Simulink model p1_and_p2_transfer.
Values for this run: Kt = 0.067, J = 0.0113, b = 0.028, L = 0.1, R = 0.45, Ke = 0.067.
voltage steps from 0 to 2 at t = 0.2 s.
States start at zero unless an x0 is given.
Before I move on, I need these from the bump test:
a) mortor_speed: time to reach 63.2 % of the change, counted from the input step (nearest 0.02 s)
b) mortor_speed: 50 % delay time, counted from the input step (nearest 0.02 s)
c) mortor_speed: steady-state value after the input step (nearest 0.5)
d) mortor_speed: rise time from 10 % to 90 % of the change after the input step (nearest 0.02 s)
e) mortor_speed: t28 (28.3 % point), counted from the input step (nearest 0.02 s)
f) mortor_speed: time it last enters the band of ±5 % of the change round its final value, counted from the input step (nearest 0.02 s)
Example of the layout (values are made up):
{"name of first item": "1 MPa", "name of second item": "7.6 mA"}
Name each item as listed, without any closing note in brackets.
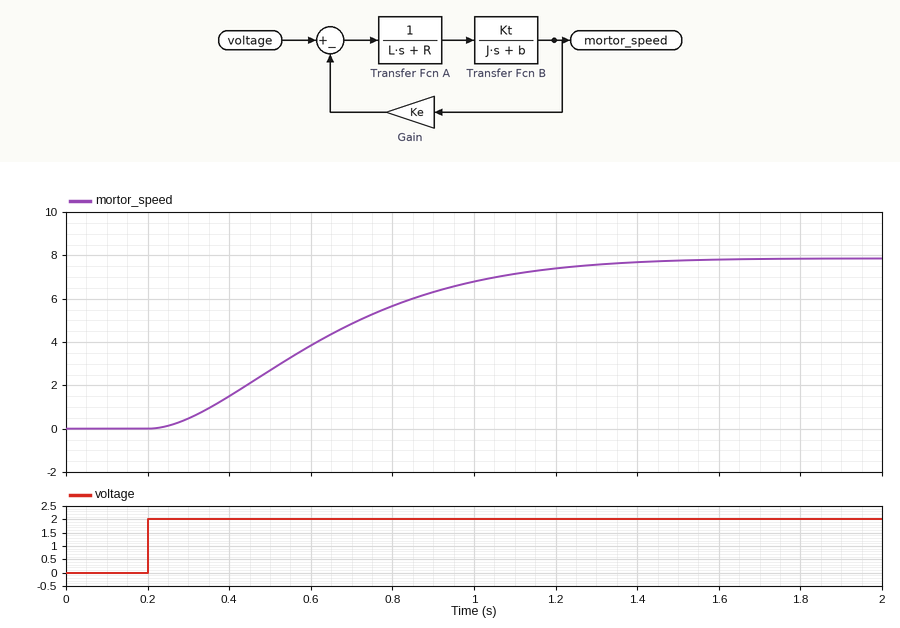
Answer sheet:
{"mortor_speed: time to reach 63.2 % of the change, counted from the input step": "0.52 s", "mortor_speed: 50 % delay time, counted from the input step": "0.40 s", "mortor_speed: steady-state value after the input step": "8.0", "mortor_speed: rise time from 10 % to 90 % of the change after the input step": "0.74 s", "mortor_speed: t28 (28.3 % point), counted from the input step": "0.26 s", "mortor_speed: time it last enters the band of ±5 % of the change round its final value, counted from the input step": "1.02 s"}
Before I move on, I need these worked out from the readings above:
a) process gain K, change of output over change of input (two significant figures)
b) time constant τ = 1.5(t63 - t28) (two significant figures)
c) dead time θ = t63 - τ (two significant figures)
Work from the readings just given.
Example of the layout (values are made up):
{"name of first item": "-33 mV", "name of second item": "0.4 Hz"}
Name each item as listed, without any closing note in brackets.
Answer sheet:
{"process gain K, change of output over change of input": "4.0", "time constant τ = 1.5(t63 - t28)": "0.39 s", "dead time θ = t63 - τ": "0.13 s"}
